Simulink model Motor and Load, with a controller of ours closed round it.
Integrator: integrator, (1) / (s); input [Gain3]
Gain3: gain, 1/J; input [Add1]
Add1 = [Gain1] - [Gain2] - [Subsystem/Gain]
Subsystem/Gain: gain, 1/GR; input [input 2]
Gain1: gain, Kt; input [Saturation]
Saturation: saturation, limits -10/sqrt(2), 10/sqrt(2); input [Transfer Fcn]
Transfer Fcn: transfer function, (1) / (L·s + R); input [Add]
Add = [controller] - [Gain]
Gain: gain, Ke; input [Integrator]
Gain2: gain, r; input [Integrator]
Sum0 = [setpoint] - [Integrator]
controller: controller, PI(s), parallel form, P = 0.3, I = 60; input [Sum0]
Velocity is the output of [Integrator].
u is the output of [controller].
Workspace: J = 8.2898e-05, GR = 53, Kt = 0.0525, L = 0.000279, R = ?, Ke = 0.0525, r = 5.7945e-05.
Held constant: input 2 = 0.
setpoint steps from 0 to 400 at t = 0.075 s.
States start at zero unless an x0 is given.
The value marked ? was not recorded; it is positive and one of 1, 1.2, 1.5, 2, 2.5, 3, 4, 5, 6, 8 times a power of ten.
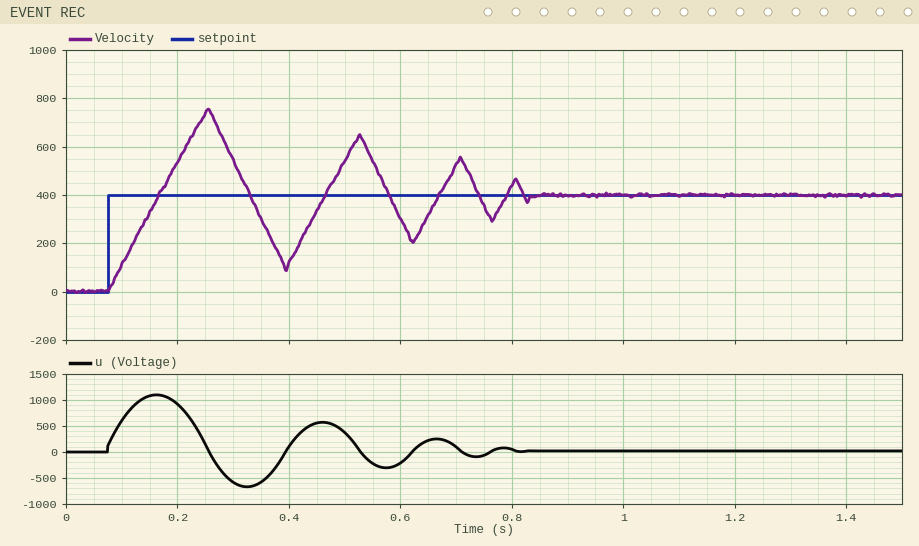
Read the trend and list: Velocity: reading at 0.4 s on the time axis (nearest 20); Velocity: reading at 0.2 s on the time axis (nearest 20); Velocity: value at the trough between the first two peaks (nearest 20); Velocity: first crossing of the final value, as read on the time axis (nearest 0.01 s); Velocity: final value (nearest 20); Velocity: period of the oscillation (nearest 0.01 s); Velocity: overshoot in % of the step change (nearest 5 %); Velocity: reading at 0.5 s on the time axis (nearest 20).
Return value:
120
540
100
0.17 s
400
0.27 s
90 %
540
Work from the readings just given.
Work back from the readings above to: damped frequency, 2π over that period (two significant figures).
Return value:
23 rad/s
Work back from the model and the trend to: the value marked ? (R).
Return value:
0.3
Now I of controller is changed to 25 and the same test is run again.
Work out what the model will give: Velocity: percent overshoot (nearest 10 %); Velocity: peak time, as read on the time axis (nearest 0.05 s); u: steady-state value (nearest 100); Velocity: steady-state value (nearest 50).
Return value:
80 %
0.25 s
0
400
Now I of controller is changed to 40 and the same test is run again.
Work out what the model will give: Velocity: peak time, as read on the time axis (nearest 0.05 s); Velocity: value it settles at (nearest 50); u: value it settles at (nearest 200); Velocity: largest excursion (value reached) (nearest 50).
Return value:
0.25 s
400
0
750
